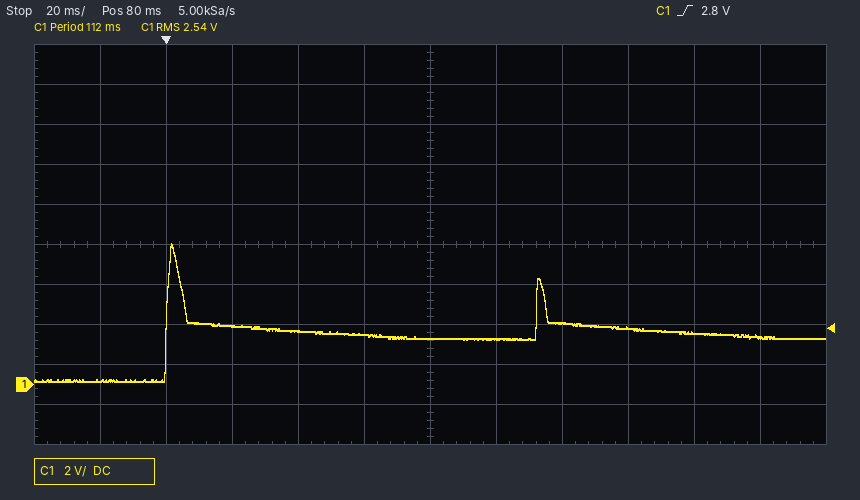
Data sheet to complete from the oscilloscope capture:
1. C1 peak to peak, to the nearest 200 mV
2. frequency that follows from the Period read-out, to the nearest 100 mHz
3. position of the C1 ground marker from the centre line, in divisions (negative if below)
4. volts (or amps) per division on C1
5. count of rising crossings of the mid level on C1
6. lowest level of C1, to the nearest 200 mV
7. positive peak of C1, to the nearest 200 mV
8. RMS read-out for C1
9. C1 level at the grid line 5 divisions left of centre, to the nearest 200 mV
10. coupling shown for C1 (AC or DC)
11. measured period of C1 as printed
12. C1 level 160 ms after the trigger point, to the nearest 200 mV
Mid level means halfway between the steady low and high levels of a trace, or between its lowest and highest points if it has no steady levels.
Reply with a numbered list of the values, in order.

1. 6.8 V
2. 8.9 Hz
3. -3.5 div
4. 2 V
5. 2
6. 200 mV
7. 7.0 V
8. 2.54 V
9. 200 mV
10. DC
11. 112 ms
12. 2.6 V
